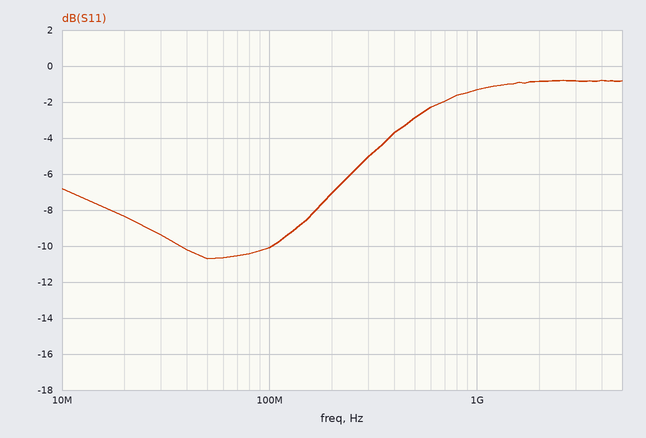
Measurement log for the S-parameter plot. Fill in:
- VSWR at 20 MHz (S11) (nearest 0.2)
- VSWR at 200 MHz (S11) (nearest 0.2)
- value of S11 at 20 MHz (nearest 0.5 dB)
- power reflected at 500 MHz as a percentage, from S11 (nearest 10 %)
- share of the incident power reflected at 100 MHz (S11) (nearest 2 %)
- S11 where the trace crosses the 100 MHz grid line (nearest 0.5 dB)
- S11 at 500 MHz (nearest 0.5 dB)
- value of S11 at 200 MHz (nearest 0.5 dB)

2.2
2.6
-8.5 dB
50 %
10 %
-10.0 dB
-3.0 dB
-7.0 dB
